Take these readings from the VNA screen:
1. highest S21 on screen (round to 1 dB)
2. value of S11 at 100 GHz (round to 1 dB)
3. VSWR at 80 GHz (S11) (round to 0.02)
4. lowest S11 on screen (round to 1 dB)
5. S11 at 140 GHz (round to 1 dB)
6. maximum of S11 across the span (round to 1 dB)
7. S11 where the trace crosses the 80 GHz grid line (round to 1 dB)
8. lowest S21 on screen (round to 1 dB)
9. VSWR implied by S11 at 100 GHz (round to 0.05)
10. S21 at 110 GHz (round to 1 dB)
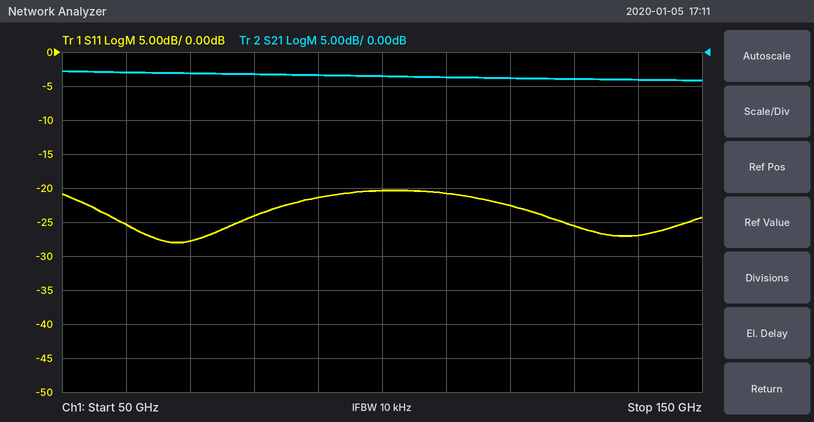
-3 dB
-20 dB
1.14
-28 dB
-27 dB
-20 dB
-24 dB
-4 dB
1.20
-4 dB
